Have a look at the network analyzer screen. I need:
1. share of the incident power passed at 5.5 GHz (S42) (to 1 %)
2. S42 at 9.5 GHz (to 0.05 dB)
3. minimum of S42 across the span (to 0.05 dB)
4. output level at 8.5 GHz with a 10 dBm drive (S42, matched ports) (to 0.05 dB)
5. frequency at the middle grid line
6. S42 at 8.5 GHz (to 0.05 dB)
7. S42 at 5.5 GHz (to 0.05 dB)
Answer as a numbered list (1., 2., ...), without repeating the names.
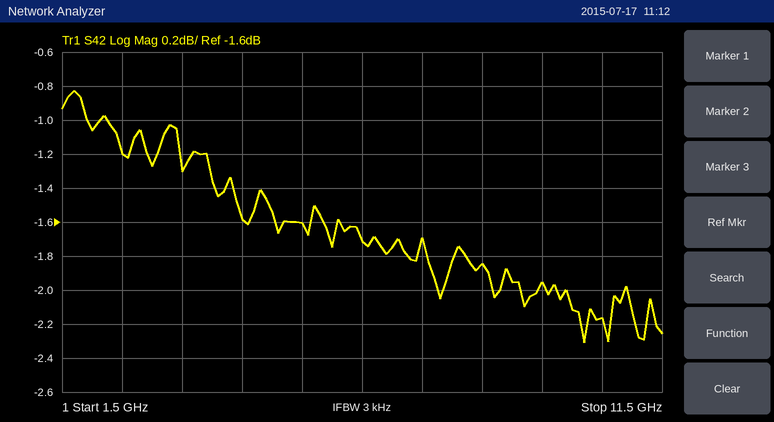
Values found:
1. 69 %
2. -1.95 dB
3. -2.30 dB
4. 8.15 dBm
5. 6.5 GHz
6. -1.85 dB
7. -1.60 dB
